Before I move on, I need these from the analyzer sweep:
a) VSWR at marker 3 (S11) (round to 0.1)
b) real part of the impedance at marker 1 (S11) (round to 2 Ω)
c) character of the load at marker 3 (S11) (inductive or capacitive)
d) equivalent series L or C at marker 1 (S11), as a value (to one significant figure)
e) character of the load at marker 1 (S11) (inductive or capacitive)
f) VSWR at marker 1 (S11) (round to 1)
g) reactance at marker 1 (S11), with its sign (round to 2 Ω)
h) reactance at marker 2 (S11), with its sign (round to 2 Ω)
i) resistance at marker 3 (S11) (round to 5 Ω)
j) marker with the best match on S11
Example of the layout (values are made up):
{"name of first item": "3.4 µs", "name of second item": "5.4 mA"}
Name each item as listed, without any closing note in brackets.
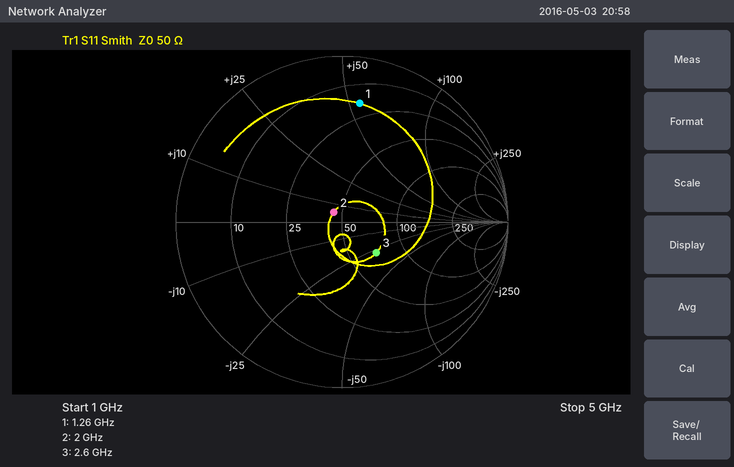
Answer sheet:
{"VSWR at marker 3 (S11)": "1.8", "real part of the impedance at marker 1 (S11)": "18 Ω", "character of the load at marker 3 (S11)": "capacitive", "equivalent series L or C at marker 1 (S11), as a value": "7 nH", "character of the load at marker 1 (S11)": "inductive", "VSWR at marker 1 (S11)": "6", "reactance at marker 1 (S11), with its sign": "+54 Ω", "reactance at marker 2 (S11), with its sign": "+6 Ω", "resistance at marker 3 (S11)": "70 Ω", "marker with the best match on S11": "marker 2"}
